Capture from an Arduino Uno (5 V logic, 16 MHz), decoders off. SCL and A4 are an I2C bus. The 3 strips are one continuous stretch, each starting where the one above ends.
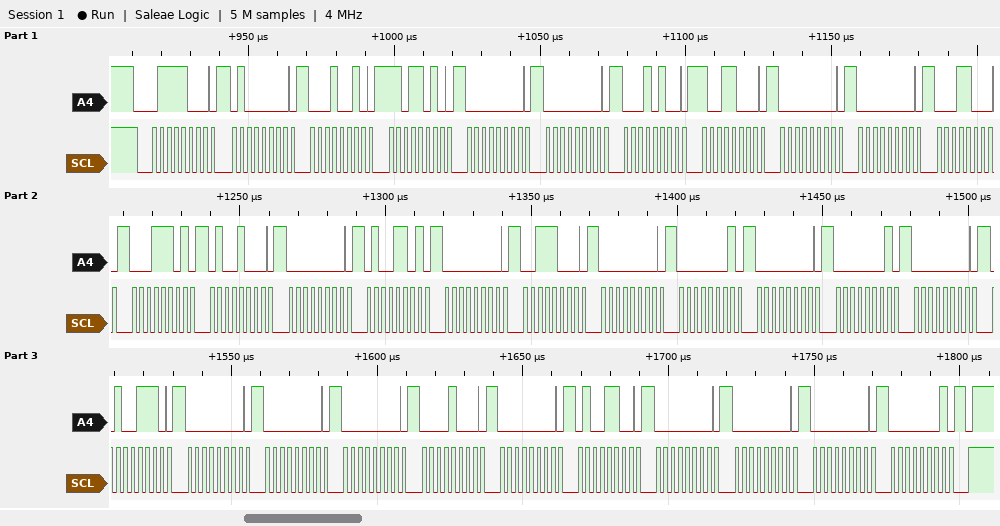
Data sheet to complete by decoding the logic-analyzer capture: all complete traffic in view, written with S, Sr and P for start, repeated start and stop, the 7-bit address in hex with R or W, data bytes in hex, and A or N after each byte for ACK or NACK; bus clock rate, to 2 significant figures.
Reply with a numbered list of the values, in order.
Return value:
1. S 3CW A 40 A 12 A DA A 00 A 00 A 14 A 98 A 00 A 00 A 18 A 1D A 48 A 00 A 4D A 00 A 38 A 00 A 01 A 00 A 01 A 00 A 4E A 00 A 00 A 00 A 08 A 00 A 4C A 00 A 00 A 00 A 01 A P
2. 400 kHz
